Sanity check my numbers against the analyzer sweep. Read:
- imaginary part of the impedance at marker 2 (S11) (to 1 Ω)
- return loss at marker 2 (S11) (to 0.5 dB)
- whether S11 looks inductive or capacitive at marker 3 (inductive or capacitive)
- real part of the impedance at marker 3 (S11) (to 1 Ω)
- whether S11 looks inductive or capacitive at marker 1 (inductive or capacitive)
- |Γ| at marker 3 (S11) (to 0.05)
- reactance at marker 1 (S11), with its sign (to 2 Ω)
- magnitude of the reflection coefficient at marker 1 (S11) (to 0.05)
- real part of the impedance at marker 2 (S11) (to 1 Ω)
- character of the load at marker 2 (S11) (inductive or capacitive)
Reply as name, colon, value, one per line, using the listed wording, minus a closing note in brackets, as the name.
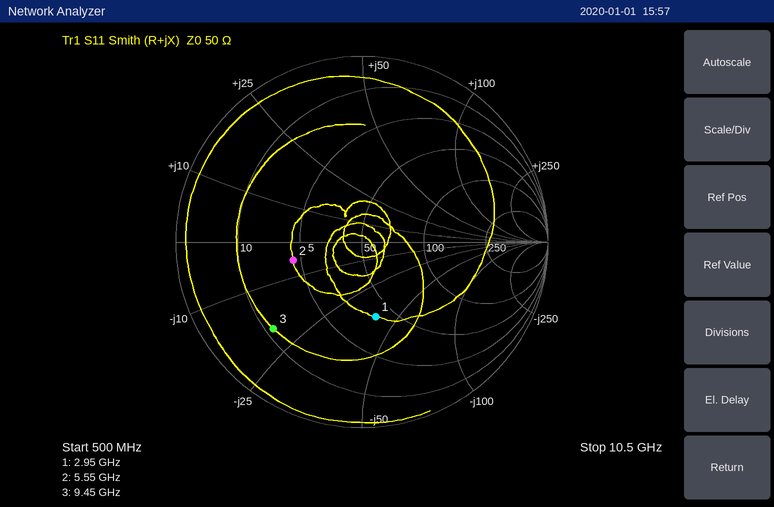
imaginary part of the impedance at marker 2 (S11): -5 Ω
return loss at marker 2 (S11): 8.5 dB
whether S11 looks inductive or capacitive at marker 3: capacitive
real part of the impedance at marker 3 (S11): 12 Ω
whether S11 looks inductive or capacitive at marker 1: capacitive
|Γ| at marker 3 (S11): 0.65
reactance at marker 1 (S11), with its sign: -40 Ω
magnitude of the reflection coefficient at marker 1 (S11): 0.40
real part of the impedance at marker 2 (S11): 23 Ω
character of the load at marker 2 (S11): capacitive
